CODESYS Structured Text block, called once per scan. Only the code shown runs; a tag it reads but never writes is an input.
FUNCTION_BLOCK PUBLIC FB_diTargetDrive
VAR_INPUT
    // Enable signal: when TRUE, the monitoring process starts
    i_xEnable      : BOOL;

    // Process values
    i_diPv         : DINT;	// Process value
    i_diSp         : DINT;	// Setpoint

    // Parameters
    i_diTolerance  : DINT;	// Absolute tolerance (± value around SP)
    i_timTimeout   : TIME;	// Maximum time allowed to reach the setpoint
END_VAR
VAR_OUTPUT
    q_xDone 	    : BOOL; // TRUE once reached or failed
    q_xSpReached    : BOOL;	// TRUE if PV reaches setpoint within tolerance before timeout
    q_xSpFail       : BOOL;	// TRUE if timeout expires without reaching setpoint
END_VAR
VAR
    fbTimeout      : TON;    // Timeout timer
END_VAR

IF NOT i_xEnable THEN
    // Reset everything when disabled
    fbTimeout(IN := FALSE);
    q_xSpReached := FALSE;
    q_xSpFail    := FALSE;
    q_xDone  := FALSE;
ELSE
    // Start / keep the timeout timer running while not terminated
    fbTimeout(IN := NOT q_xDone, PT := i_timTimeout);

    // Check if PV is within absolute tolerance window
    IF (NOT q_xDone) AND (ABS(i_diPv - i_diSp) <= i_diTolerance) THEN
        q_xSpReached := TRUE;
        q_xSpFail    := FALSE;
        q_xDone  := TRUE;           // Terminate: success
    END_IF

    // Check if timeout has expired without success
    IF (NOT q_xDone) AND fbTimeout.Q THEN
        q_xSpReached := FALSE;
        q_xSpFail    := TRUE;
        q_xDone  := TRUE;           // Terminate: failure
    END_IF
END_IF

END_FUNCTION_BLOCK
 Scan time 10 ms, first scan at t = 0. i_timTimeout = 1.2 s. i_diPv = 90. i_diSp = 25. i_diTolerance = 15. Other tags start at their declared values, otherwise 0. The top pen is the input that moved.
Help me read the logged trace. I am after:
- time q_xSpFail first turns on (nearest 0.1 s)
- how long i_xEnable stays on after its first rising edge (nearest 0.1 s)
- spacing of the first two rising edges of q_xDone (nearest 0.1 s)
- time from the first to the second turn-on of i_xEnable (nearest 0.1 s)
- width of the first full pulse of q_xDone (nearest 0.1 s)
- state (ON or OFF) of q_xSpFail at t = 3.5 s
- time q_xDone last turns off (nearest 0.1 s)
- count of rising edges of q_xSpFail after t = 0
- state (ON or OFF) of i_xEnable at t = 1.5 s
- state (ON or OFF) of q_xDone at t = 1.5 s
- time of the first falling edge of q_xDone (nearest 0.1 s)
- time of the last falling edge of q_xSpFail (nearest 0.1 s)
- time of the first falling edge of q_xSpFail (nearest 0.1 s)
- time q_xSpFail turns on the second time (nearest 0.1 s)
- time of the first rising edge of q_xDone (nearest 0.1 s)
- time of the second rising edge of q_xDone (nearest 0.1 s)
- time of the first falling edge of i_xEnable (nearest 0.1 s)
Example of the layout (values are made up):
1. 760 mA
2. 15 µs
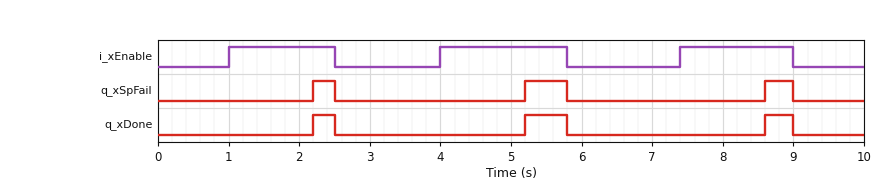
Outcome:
1. 2.2 s
2. 1.5 s
3. 3.0 s
4. 3.0 s
5. 0.3 s
6. OFF
7. 9.0 s
8. 3
9. ON
10. OFF
11. 2.5 s
12. 9.0 s
13. 2.5 s
14. 5.2 s
15. 2.2 s
16. 5.2 s
17. 2.5 s
